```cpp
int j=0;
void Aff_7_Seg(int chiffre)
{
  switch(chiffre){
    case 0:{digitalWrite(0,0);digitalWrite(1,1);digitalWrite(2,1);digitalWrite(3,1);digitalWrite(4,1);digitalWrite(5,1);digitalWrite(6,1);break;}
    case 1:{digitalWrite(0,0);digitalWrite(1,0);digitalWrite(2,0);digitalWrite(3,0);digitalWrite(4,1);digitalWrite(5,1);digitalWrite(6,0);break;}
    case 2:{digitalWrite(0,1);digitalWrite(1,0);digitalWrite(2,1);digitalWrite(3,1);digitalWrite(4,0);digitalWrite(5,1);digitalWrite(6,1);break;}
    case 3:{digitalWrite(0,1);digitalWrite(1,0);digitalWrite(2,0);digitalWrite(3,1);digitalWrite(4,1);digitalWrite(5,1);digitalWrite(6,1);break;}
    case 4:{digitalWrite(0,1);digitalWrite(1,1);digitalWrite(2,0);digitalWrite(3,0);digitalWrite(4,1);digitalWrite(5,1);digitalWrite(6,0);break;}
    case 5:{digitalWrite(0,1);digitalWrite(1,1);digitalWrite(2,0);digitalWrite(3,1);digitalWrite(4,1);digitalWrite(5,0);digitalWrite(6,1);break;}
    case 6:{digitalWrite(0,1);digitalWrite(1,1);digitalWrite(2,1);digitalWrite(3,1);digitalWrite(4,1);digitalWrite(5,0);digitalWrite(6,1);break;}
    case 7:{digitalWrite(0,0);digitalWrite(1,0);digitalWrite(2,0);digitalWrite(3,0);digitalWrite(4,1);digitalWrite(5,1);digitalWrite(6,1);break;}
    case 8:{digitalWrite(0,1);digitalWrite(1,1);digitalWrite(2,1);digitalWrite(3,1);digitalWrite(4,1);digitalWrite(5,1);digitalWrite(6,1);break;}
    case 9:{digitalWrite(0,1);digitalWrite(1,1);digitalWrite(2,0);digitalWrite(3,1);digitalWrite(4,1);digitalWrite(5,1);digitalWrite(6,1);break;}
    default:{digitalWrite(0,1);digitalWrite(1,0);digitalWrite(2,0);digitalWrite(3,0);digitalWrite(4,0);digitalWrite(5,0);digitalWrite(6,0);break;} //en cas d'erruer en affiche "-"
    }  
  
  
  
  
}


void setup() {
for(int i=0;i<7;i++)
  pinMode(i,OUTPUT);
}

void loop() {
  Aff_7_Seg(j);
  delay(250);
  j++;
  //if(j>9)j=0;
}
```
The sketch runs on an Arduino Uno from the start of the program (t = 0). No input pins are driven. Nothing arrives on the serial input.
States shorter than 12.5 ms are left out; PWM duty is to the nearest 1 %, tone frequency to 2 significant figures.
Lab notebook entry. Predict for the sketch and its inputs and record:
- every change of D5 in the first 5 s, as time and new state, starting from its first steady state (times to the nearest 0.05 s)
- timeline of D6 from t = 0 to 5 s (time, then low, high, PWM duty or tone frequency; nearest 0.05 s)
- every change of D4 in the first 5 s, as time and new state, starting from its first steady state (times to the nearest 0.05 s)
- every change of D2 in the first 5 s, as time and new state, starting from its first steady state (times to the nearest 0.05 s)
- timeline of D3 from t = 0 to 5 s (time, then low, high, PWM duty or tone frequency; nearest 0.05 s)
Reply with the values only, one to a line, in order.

0 s high; 1.25 s low; 1.75 s high; 2.5 s low
0 s high; 0.25 s low; 0.5 s high; 1 s low; 1.25 s high; 2.5 s low
0 s high; 0.5 s low; 0.75 s high; 2.5 s low
0 s high; 0.25 s low; 0.5 s high; 0.75 s low; 1.5 s high; 1.75 s low; 2 s high; 2.25 s low
0 s high; 0.25 s low; 0.5 s high; 1 s low; 1.25 s high; 1.75 s low; 2 s high; 2.5 s low
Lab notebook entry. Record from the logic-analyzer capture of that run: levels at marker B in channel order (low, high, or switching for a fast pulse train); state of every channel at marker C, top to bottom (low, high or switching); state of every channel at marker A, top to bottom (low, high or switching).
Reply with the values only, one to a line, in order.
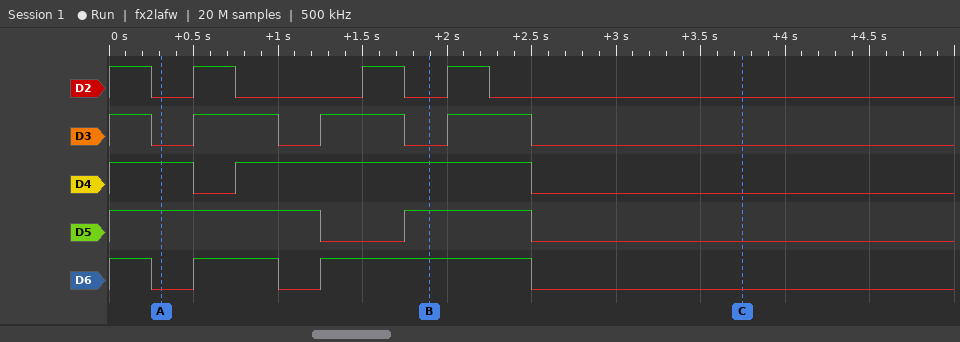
D2 low, D3 low, D4 high, D5 high, D6 high
D2 low, D3 low, D4 low, D5 low, D6 low
D2 low, D3 low, D4 high, D5 high, D6 low
